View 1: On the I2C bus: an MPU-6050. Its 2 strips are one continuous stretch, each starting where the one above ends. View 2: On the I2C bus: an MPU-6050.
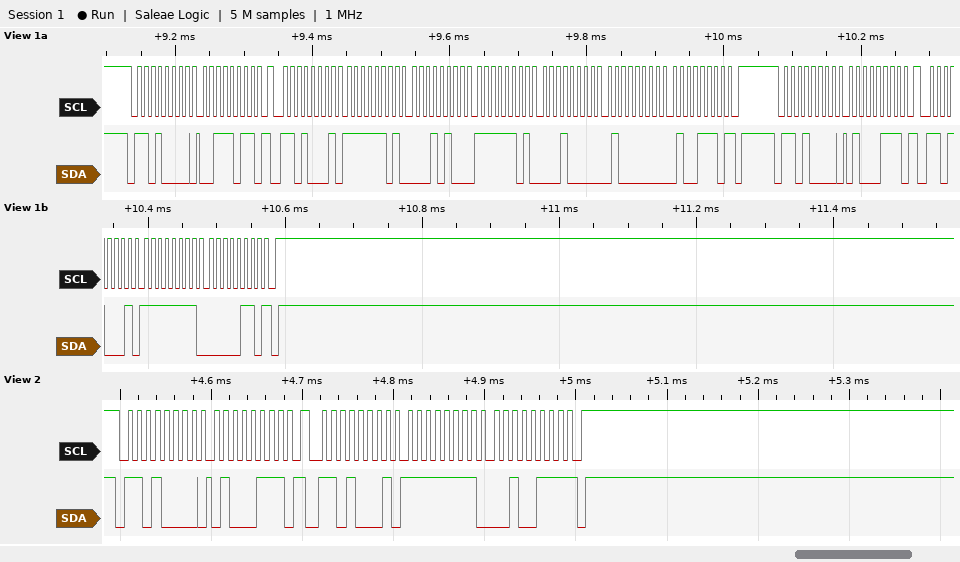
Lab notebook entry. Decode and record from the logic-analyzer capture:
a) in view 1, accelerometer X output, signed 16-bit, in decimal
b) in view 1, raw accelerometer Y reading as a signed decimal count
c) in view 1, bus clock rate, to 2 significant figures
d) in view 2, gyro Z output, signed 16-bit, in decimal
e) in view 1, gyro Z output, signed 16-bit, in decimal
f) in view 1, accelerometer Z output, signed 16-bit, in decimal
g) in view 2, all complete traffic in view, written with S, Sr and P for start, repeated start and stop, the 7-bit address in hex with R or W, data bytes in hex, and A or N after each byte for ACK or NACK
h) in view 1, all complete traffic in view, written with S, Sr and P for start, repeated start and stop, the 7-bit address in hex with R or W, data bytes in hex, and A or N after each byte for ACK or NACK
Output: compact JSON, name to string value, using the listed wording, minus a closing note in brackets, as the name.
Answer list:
{"in view 1, accelerometer X output, signed 16-bit, in decimal": "-748", "in view 1, raw accelerometer Y reading as a signed decimal count": "-752", "in view 1, bus clock rate, to 2 significant figures": "100 kHz", "in view 2, gyro Z output, signed 16-bit, in decimal": "-217", "in view 1, gyro Z output, signed 16-bit, in decimal": "-250", "in view 1, accelerometer Z output, signed 16-bit, in decimal": "16462", "in view 2, all complete traffic in view, written with S, Sr and P for start, repeated start and stop, the 7-bit address in hex with R or W, data bytes in hex, and A or N after each byte for ACK or NACK": "S 68W A 47 A Sr 68R A FF A 27 N P", "in view 1, all complete traffic in view, written with S, Sr and P for start, repeated start and stop, the 7-bit address in hex with R or W, data bytes in hex, and A or N after each byte for ACK or NACK": "S 68W A 3B A Sr 68R A FD A 14 A FD A 10 A 40 A 4E N P S 68W A 47 A Sr 68R A FF A 06 N P"}
